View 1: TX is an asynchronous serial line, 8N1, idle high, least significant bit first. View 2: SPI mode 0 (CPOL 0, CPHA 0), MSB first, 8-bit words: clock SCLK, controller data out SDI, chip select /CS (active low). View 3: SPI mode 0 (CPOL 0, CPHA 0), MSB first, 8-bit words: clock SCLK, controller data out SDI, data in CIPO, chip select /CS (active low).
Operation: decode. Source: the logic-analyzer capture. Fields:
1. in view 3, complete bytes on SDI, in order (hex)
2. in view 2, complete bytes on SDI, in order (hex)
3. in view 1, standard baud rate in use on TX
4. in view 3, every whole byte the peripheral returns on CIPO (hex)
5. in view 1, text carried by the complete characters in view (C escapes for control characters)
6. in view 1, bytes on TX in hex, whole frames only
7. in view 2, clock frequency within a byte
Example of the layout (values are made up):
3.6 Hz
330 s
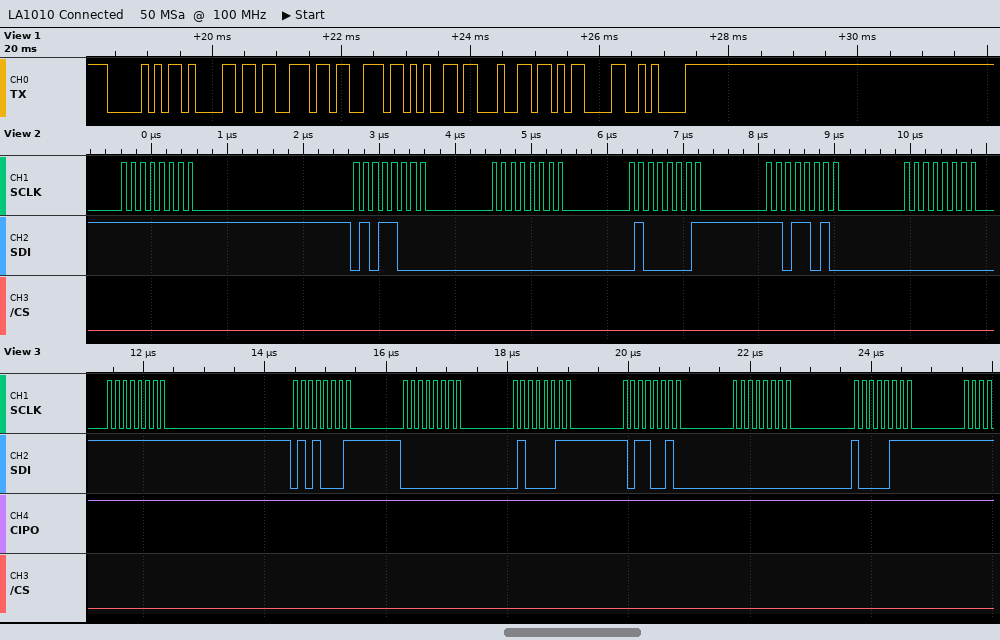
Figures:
FF 51 00 43 B2 00 87
0xFF 0x58 0x00 0x41 0xDA 0x00
9600 baud
FF FF FF FF FF FF FF
"Passed\r\n"
50 61 73 73 65 64 0D 0A
8 MHz
